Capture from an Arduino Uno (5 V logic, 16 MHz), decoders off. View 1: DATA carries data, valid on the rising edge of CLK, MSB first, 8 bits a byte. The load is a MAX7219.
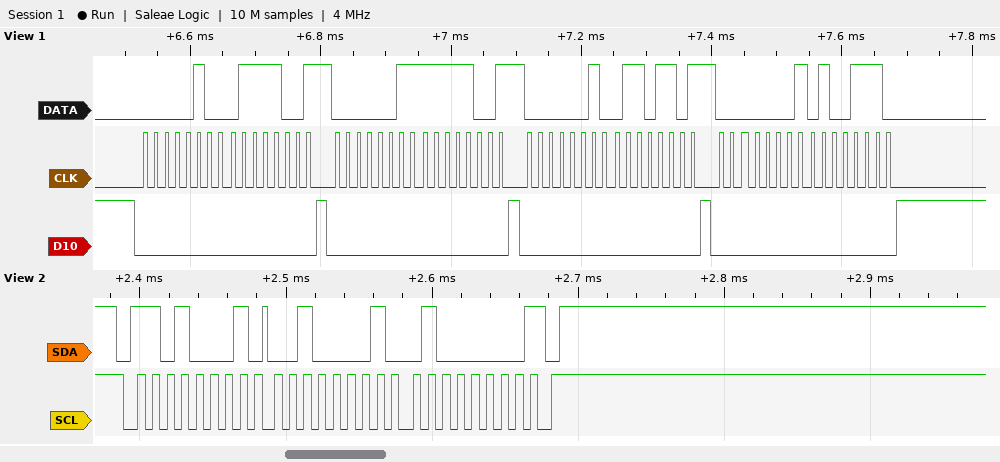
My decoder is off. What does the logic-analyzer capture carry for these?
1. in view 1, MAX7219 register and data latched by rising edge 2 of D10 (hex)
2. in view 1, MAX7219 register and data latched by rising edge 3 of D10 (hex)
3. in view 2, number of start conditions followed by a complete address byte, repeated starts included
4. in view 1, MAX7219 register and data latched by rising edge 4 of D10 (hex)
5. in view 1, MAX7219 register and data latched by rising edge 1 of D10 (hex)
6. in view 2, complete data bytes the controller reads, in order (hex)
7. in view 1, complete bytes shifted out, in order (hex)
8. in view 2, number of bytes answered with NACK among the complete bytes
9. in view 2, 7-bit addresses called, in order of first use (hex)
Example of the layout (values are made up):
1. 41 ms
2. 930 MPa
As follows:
1. register 0x3, data 0xF9
2. register 0x2, data 0x6D
3. 1
4. register 0x1, data 0x4E
5. register 0x4, data 0x79
6. 21 40
7. 0x04 0x79 0x03 0xF9 0x02 0x6D 0x01 0x4E
8. 1
9. 0x68
